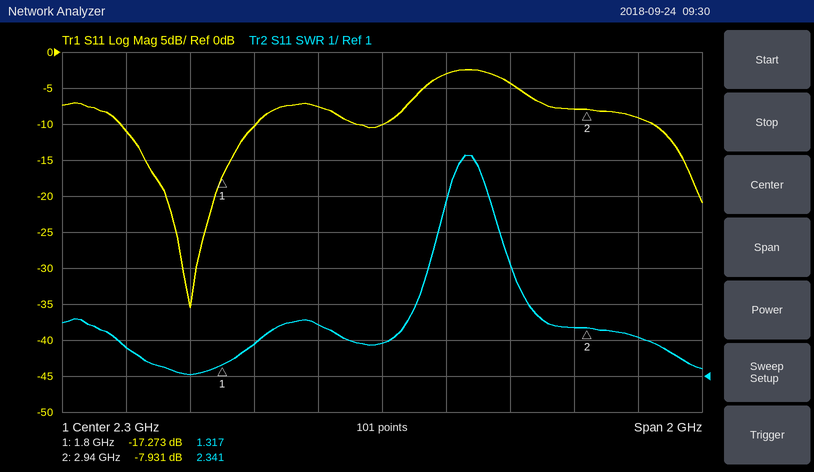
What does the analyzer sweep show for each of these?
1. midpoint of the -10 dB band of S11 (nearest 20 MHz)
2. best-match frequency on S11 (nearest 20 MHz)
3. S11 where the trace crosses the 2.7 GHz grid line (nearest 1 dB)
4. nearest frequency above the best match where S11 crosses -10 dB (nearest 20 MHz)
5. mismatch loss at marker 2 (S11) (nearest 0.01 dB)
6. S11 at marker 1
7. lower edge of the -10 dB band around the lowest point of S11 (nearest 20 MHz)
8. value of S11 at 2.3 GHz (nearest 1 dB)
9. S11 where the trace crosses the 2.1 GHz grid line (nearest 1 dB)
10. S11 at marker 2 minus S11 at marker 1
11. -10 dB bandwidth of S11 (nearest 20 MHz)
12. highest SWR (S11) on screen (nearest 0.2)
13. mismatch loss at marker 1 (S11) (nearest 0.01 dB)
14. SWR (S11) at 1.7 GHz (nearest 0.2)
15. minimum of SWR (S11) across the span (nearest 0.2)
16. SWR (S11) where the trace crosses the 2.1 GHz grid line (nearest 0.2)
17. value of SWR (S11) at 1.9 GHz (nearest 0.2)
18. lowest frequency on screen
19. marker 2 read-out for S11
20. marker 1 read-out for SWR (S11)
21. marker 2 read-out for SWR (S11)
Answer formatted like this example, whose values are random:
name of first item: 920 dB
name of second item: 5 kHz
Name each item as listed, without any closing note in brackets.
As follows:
midpoint of the -10 dB band of S11: 1.70 GHz
best-match frequency on S11: 1.70 GHz
S11 where the trace crosses the 2.7 GHz grid line: -4 dB
nearest frequency above the best match where S11 crosses -10 dB: 1.90 GHz
mismatch loss at marker 2 (S11): 0.76 dB
S11 at marker 1: -17.273 dB
lower edge of the -10 dB band around the lowest point of S11: 1.48 GHz
value of S11 at 2.3 GHz: -10 dB
S11 where the trace crosses the 2.1 GHz grid line: -8 dB
S11 at marker 2 minus S11 at marker 1: 9.342 dB
-10 dB bandwidth of S11: 420 MHz
highest SWR (S11) on screen: 7.2
mismatch loss at marker 1 (S11): 0.08 dB
SWR (S11) at 1.7 GHz: 1.0
minimum of SWR (S11) across the span: 1.0
SWR (S11) where the trace crosses the 2.1 GHz grid line: 2.4
value of SWR (S11) at 1.9 GHz: 1.8
lowest frequency on screen: 1.3 GHz
marker 2 read-out for S11: -7.931 dB
marker 1 read-out for SWR: 1.317
marker 2 read-out for SWR: 2.341
